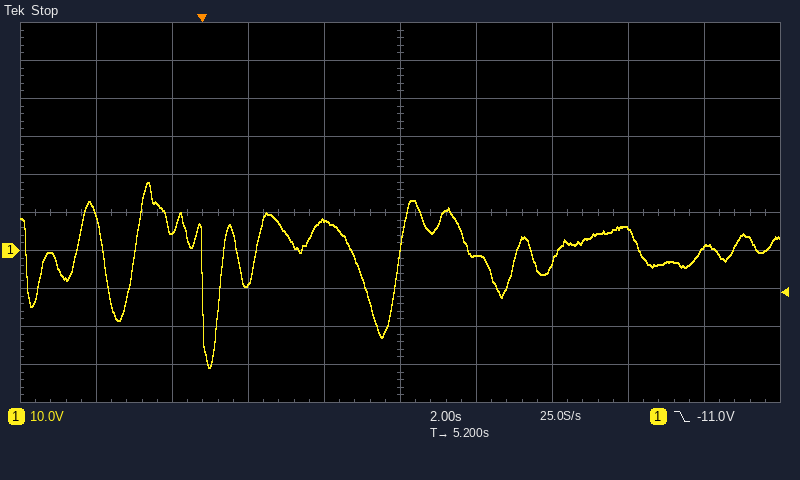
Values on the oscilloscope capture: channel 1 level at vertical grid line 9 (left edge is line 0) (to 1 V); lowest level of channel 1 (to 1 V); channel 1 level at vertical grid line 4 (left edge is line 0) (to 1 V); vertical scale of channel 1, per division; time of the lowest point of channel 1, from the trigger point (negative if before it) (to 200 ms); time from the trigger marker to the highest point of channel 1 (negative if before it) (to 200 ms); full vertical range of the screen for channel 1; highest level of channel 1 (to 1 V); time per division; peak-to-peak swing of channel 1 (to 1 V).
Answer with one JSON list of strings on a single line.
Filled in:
["1 V", "-31 V", "8 V", "10 V", "+200 ms", "-1.4 s", "100 V", "18 V", "2 s", "49 V"]
